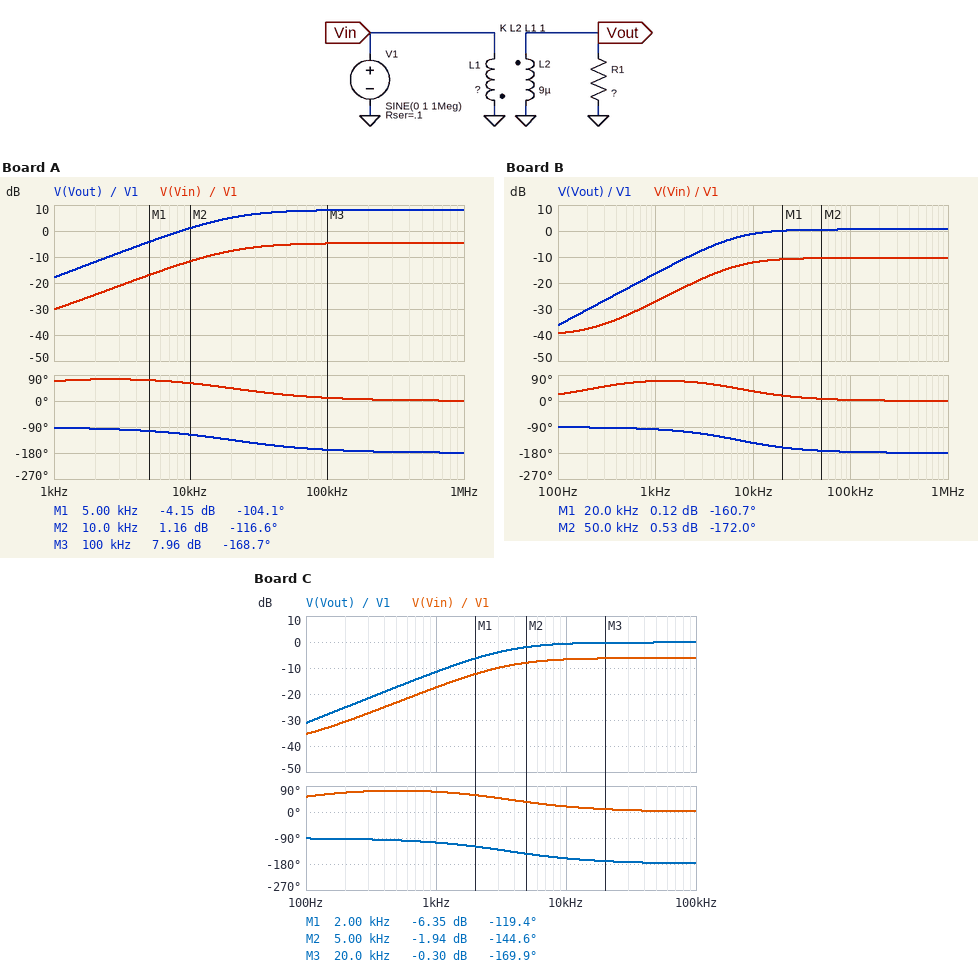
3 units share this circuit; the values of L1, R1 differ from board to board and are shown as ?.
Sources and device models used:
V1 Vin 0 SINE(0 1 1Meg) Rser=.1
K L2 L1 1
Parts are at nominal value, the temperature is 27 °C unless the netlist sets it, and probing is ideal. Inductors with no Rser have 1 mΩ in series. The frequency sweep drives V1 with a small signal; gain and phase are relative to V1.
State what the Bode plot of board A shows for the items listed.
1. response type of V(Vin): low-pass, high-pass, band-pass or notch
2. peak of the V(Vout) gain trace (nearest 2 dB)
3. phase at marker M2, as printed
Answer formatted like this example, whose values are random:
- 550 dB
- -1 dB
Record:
- high-pass
- 8 dB
- -116.6 deg
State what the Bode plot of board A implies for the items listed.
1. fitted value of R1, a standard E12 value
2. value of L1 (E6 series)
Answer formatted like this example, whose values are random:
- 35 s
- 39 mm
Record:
- 2.7 Ω
- 470 nH
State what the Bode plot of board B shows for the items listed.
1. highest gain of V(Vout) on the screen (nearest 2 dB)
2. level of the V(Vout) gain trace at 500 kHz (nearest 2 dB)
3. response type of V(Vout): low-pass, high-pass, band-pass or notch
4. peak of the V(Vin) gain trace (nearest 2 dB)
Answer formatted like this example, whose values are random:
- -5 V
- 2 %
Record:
- 0 dB
- 0 dB
- high-pass
- -10 dB
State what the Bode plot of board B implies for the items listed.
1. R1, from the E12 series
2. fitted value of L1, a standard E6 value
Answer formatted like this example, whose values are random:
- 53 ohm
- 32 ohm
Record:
- 0.56 Ω
- 680 nH
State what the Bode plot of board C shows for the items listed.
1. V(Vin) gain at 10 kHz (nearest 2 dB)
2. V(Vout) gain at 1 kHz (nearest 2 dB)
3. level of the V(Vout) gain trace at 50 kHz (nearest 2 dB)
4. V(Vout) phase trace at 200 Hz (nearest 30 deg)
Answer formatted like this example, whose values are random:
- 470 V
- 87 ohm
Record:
- -6 dB
- -12 dB
- 0 dB
- -90 deg
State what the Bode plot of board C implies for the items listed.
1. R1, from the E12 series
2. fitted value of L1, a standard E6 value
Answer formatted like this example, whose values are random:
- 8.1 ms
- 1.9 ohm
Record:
- 0.39 Ω
- 2.2 µH
